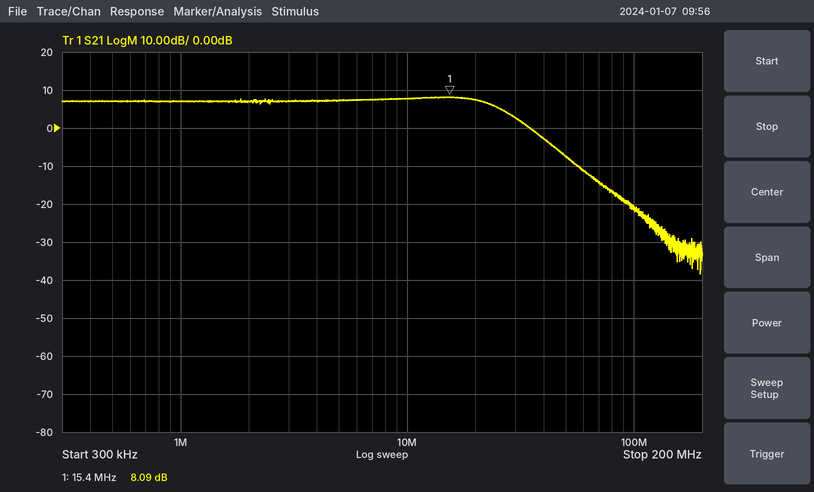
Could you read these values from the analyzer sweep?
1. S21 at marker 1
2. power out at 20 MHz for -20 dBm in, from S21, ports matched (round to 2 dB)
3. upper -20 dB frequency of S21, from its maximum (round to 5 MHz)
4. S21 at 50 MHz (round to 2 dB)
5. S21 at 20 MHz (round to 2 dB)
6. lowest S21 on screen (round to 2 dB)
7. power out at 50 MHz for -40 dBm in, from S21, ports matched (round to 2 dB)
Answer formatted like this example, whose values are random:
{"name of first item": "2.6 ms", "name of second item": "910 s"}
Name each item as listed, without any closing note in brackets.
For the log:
{"S21 at marker 1": "8.09 dB", "power out at 20 MHz for -20 dBm in, from S21, ports matched": "-12 dBm", "upper -20 dB frequency of S21, from its maximum": "60 MHz", "S21 at 50 MHz": "-8 dB", "S21 at 20 MHz": "8 dB", "lowest S21 on screen": "-38 dB", "power out at 50 MHz for -40 dBm in, from S21, ports matched": "-48 dBm"}
